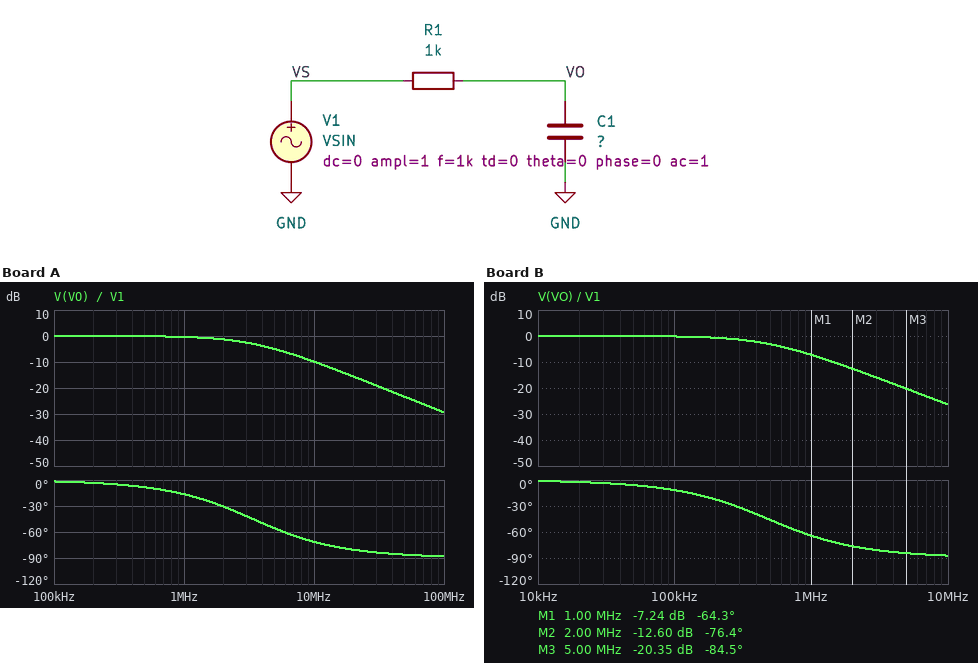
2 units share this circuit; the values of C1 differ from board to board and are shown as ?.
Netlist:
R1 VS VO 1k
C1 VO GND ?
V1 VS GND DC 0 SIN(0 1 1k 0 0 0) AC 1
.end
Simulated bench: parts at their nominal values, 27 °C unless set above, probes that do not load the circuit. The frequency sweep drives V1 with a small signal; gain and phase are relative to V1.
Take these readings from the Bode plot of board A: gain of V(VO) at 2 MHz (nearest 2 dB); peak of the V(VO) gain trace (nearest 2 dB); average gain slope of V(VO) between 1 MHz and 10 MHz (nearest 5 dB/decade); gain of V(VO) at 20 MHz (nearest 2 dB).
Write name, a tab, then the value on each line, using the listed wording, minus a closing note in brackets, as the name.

gain of V(VO) at 2 MHz	-2 dB
peak of the V(VO) gain trace	0 dB
average gain slope of V(VO) between 1 MHz and 10 MHz	-10 dB/decade
gain of V(VO) at 20 MHz	-16 dB
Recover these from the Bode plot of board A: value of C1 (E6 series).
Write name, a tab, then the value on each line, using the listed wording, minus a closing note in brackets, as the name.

value of C1	47 pF
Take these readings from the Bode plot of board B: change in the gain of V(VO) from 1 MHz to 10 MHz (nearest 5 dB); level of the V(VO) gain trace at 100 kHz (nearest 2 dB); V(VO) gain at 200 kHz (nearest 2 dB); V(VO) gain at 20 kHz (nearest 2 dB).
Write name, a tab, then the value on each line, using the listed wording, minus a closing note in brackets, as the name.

change in the gain of V(VO) from 1 MHz to 10 MHz	-20 dB
level of the V(VO) gain trace at 100 kHz	0 dB
V(VO) gain at 200 kHz	0 dB
V(VO) gain at 20 kHz	0 dB
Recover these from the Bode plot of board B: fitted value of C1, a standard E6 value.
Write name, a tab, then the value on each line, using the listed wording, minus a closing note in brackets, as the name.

fitted value of C1, a standard E6 value	330 pF
